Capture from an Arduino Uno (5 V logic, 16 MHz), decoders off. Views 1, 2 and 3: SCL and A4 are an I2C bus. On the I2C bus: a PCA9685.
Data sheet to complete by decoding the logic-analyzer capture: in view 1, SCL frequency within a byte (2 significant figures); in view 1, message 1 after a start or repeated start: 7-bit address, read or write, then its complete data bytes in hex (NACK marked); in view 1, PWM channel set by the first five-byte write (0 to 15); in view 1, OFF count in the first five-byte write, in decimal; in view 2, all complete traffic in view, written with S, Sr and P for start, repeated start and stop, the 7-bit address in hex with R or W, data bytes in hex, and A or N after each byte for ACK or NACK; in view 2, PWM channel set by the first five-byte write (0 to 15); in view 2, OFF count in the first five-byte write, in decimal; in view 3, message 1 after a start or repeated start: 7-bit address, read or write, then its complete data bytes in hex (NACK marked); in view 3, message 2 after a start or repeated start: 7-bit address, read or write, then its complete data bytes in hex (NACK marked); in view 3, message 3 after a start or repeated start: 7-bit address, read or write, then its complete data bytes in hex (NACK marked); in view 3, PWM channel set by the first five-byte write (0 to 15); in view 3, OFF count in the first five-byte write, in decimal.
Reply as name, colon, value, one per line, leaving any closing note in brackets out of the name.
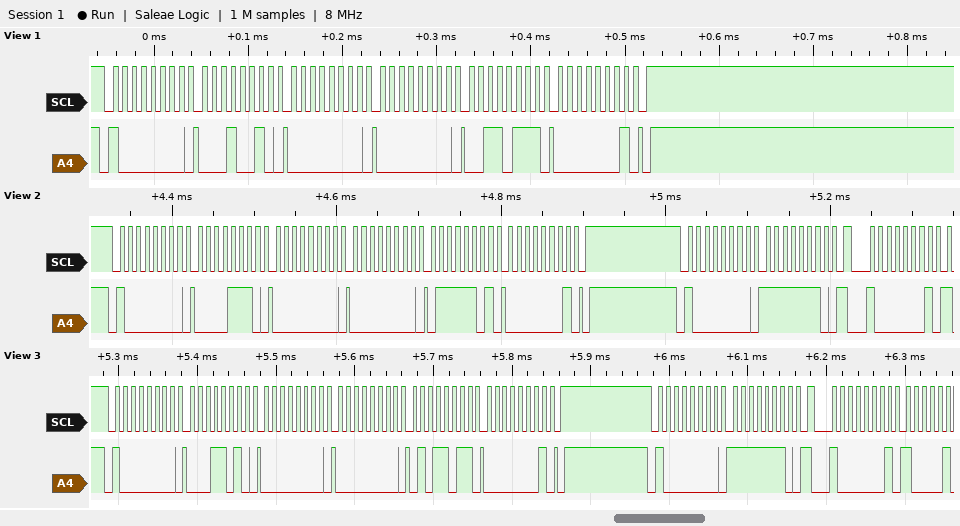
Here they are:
in view 1, SCL frequency within a byte: 100 kHz
in view 1, message 1 after a start or repeated start: 7-bit address, read or write, then its complete data bytes in hex: 0x40 write: 12 00 00 37 01
in view 1, PWM channel set by the first five-byte write: 3
in view 1, OFF count in the first five-byte write, in decimal: 311
in view 2, all complete traffic in view, written with S, Sr and P for start, repeated start and stop, the 7-bit address in hex with R or W, data bytes in hex, and A or N after each byte for ACK or NACK: S 40W A 0E A 00 A 00 A 7D A 01 A P S 40W A FE A Sr 40R A
in view 2, PWM channel set by the first five-byte write: 2
in view 2, OFF count in the first five-byte write, in decimal: 381
in view 3, message 1 after a start or repeated start: 7-bit address, read or write, then its complete data bytes in hex: 0x40 write: 1A 00 00 5B 01
in view 3, message 2 after a start or repeated start: 7-bit address, read or write, then its complete data bytes in hex: 0x40 write: FE
in view 3, message 3 after a start or repeated start: 7-bit address, read or write, then its complete data bytes in hex: 0x40 read
in view 3, PWM channel set by the first five-byte write: 5
in view 3, OFF count in the first five-byte write, in decimal: 347
